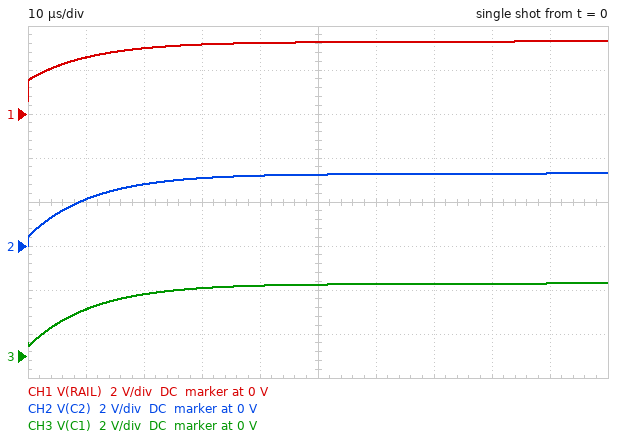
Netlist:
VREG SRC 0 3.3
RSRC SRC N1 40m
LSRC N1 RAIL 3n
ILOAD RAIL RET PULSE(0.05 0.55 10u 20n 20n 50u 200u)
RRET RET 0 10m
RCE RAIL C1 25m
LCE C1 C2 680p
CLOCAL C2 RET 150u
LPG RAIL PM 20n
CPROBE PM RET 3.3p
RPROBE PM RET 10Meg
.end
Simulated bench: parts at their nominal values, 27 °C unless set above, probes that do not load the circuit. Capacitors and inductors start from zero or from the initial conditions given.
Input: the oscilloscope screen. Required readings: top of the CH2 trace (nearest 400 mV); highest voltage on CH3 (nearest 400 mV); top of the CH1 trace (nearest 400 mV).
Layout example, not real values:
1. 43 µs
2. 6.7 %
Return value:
1. 3.2 V
2. 3.2 V
3. 3.2 V
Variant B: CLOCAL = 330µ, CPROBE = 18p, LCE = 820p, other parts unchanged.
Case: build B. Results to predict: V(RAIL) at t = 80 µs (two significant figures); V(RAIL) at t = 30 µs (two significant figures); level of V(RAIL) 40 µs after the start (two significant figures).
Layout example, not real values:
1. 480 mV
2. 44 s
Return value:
1. 3.2 V
2. 2.8 V
3. 2.9 V
